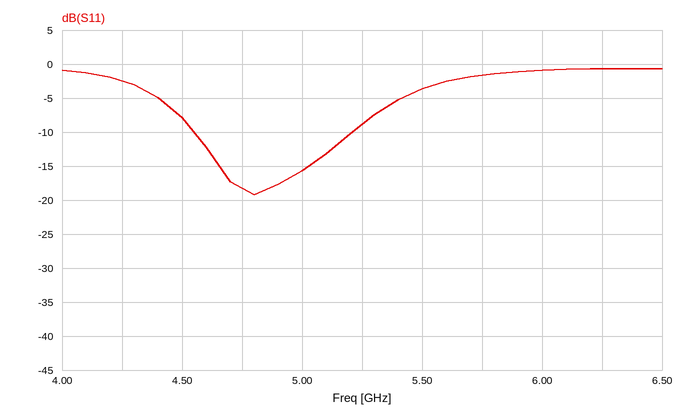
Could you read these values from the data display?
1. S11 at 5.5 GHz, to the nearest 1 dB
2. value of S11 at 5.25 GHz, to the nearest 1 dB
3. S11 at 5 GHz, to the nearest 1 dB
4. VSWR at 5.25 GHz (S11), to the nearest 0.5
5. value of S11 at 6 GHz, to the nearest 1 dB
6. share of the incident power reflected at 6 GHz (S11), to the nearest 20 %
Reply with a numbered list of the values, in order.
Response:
1. -4 dB
2. -9 dB
3. -16 dB
4. 2.0
5. -1 dB
6. 80 %
